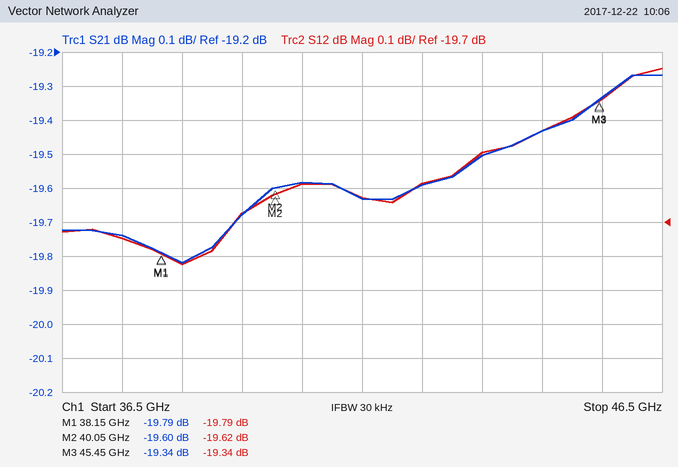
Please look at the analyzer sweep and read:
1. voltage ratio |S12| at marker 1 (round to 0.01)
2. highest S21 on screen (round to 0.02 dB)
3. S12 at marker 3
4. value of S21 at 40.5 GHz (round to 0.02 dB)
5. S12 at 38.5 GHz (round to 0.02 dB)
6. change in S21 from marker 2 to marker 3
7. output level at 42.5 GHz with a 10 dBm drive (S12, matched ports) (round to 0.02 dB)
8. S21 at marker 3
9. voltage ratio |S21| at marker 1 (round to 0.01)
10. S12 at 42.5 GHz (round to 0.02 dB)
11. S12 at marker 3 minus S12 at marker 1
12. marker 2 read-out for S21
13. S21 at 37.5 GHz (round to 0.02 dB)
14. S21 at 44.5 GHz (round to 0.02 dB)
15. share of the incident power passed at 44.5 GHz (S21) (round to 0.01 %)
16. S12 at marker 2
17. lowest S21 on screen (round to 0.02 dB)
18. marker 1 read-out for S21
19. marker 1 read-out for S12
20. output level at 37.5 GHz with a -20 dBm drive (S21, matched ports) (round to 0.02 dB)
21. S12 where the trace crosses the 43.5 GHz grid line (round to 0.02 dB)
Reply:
0.10
-19.26 dB
-19.34 dB
-19.58 dB
-19.82 dB
0.26 dB
-9.58 dBm
-19.34 dB
0.10
-19.58 dB
0.45 dB
-19.60 dB
-19.74 dB
-19.44 dB
1.14 %
-19.62 dB
-19.82 dB
-19.79 dB
-19.79 dB
-39.74 dBm
-19.50 dB
